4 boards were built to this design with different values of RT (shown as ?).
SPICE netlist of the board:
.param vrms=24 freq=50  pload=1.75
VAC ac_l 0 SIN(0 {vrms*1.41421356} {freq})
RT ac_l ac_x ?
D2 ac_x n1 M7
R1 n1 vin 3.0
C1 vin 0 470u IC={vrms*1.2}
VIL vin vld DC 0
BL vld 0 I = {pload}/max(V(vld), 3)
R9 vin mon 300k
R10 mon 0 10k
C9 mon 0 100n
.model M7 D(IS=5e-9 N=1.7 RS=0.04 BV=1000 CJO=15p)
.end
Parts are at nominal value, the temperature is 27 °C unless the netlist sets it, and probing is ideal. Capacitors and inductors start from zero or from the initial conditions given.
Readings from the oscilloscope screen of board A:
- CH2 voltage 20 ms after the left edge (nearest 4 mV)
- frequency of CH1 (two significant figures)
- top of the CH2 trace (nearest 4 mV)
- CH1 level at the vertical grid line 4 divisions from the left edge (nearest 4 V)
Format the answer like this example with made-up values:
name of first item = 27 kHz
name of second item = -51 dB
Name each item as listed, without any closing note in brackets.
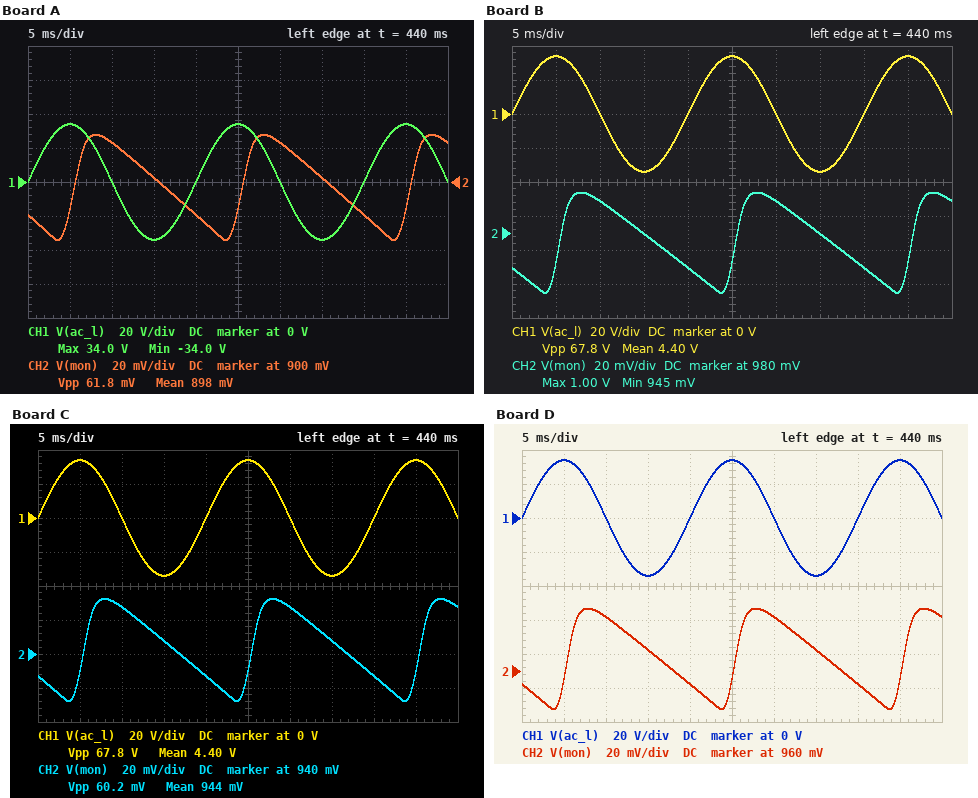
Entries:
CH2 voltage 20 ms after the left edge = 880 mV
frequency of CH1 = 50 Hz
top of the CH2 trace = 928 mV
CH1 level at the vertical grid line 4 divisions from the left edge = 0 V
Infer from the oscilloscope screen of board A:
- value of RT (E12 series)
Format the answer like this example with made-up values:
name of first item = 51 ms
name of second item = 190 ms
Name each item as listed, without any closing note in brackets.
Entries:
value of RT = 6.8 Ω
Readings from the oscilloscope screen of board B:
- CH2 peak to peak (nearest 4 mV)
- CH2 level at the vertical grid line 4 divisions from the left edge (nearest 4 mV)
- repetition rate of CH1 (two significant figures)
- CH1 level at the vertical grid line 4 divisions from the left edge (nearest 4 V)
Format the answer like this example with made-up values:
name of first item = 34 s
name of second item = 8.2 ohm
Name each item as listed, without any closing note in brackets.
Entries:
CH2 peak to peak = 60 mV
CH2 level at the vertical grid line 4 divisions from the left edge = 960 mV
repetition rate of CH1 = 50 Hz
CH1 level at the vertical grid line 4 divisions from the left edge = 0 V
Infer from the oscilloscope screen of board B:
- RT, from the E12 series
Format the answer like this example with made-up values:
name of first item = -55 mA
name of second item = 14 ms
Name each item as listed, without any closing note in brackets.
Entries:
RT, from the E12 series = 1 Ω
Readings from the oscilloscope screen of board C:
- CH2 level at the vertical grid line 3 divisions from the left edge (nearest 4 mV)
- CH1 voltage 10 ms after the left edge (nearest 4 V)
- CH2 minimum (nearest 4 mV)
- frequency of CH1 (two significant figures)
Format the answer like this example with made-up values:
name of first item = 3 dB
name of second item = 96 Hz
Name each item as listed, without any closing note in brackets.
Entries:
CH2 level at the vertical grid line 3 divisions from the left edge = 948 mV
CH1 voltage 10 ms after the left edge = 0 V
CH2 minimum = 912 mV
frequency of CH1 = 50 Hz
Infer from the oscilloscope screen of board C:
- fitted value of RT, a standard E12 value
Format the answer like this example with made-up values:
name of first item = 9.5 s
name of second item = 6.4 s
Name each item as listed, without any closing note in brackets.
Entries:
fitted value of RT, a standard E12 value = 3.3 Ω
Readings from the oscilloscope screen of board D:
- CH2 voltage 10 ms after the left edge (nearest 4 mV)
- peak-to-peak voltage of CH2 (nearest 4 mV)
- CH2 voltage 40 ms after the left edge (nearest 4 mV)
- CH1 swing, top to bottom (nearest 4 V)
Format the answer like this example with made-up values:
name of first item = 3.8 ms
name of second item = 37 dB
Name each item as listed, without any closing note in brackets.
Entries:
CH2 voltage 10 ms after the left edge = 992 mV
peak-to-peak voltage of CH2 = 60 mV
CH2 voltage 40 ms after the left edge = 952 mV
CH1 swing, top to bottom = 68 V
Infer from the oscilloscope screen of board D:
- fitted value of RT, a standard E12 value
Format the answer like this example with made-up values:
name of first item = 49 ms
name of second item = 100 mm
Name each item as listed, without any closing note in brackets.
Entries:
fitted value of RT, a standard E12 value = 1.5 Ω
